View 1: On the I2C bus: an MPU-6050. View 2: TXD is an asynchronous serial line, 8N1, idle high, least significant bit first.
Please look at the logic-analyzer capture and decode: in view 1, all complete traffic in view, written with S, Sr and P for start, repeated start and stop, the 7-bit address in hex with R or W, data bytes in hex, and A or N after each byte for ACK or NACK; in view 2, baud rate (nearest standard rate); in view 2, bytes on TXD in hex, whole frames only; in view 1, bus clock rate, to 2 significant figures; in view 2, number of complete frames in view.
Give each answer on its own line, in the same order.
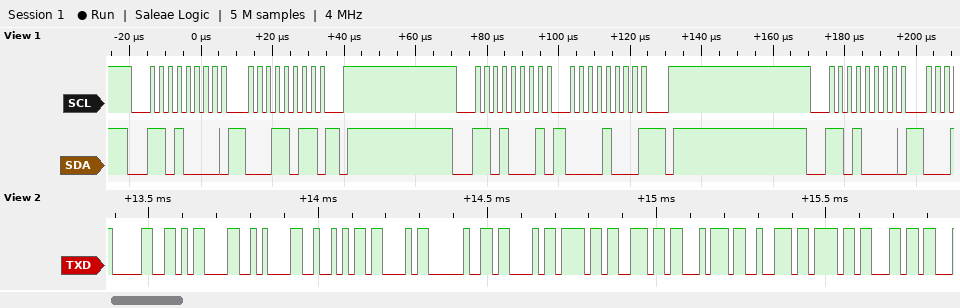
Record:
S 68W A 1B A P S 68R A 08 N P S 68W A
57600 baud
0x30 0x0D 0x0A 0x52 0x43 0x20 0x43 0x6F 0x6E 0x74 0x72 0x6F 0x6C
400 kHz
13
